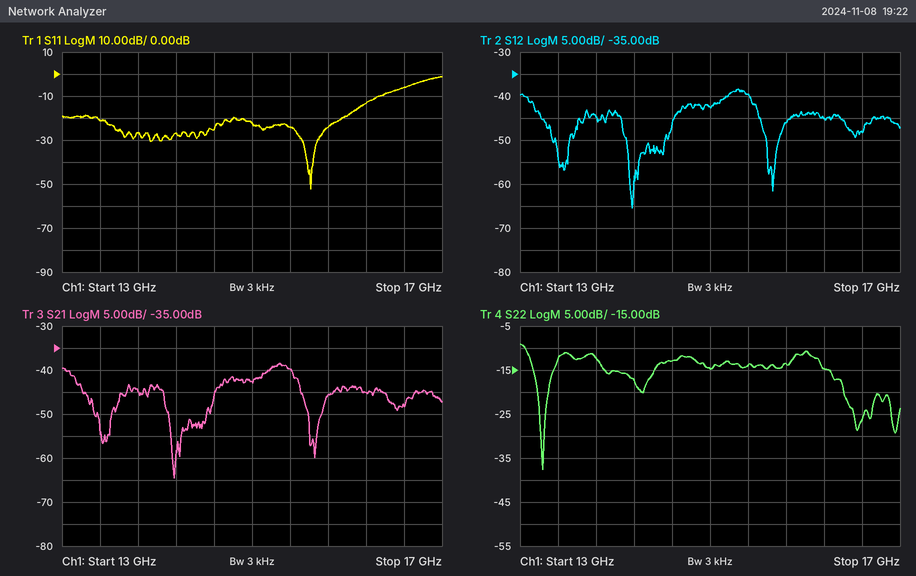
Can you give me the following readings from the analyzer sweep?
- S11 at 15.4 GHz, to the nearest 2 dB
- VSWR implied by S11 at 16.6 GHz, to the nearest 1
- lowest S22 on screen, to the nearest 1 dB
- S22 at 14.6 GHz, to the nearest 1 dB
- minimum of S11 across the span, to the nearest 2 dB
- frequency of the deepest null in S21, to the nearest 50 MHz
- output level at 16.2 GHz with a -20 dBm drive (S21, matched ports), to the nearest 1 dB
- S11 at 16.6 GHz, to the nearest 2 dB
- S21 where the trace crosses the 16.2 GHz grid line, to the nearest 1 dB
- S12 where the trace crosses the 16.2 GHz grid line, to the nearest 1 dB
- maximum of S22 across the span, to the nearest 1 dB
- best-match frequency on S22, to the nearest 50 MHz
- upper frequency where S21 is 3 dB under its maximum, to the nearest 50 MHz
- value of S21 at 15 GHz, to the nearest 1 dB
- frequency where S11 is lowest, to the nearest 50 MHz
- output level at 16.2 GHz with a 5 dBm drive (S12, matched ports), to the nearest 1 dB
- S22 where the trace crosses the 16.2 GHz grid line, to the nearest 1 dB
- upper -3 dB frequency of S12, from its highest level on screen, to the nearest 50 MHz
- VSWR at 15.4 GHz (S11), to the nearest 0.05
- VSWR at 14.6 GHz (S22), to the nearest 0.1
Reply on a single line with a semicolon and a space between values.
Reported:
-24 dB; 3; -38 dB; -13 dB; -52 dB; 14.20 GHz; -65 dBm; -6 dB; -45 dB; -45 dB; -9 dB; 13.25 GHz; 15.45 GHz; -43 dB; 15.60 GHz; -40 dBm; -15 dB; 15.45 GHz; 1.15; 1.6
